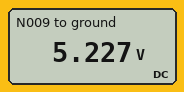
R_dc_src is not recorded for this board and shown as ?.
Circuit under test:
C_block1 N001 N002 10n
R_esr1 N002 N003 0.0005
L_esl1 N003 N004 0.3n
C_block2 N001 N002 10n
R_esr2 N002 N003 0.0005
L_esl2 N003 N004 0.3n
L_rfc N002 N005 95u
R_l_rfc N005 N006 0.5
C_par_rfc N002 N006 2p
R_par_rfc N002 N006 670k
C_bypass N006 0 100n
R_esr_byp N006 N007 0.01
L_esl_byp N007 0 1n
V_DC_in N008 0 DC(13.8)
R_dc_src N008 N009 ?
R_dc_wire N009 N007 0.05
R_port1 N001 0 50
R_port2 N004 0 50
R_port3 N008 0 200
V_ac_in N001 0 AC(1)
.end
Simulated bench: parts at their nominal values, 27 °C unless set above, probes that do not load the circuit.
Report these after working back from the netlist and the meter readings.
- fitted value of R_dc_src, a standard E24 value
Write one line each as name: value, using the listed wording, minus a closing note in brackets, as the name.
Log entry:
fitted value of R_dc_src, a standard E24 value: 0.082 Ω
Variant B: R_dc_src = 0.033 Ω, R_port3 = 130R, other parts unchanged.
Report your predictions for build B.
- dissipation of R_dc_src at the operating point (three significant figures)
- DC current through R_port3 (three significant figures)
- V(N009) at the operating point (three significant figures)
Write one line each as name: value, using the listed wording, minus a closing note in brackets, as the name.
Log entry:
dissipation of R_dc_src at the operating point: 912 W
DC current through R_port3: 106 mA
V(N009) at the operating point: 8.31 V
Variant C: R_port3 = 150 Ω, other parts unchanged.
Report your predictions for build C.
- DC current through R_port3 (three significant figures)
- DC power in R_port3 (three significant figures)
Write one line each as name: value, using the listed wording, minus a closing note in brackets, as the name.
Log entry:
DC current through R_port3: 92.0 mA
DC power in R_port3: 1.27 W
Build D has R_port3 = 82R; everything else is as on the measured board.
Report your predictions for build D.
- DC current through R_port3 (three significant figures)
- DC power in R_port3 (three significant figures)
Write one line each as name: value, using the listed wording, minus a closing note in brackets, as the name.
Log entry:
DC current through R_port3: 168 mA
DC power in R_port3: 2.32 W
